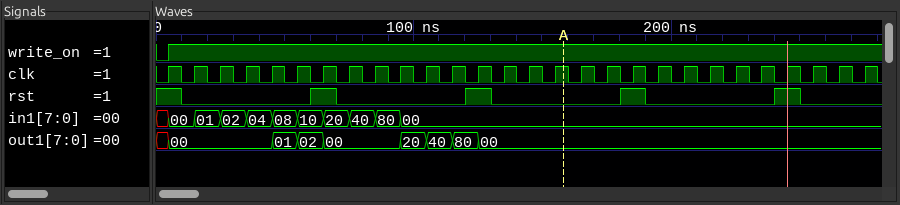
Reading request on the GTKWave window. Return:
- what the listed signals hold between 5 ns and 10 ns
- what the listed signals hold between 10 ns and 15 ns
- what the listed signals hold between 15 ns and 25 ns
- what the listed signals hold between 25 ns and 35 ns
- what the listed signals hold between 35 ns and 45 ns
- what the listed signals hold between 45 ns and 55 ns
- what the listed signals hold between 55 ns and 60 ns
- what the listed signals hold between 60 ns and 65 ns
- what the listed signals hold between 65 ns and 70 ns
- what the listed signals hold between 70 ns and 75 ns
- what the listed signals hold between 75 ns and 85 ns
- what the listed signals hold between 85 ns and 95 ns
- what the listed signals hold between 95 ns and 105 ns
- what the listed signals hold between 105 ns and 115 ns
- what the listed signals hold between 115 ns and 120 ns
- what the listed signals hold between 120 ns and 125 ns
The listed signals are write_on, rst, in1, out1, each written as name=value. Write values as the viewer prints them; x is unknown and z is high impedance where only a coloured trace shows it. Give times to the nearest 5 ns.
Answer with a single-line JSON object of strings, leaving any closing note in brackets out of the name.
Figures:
{"what the listed signals hold between 5 ns and 10 ns": "write_on=1, rst=1, in1=00, out1=00", "what the listed signals hold between 10 ns and 15 ns": "write_on=1, rst=0, in1=00, out1=00", "what the listed signals hold between 15 ns and 25 ns": "write_on=1, rst=0, in1=01, out1=00", "what the listed signals hold between 25 ns and 35 ns": "write_on=1, rst=0, in1=02, out1=00", "what the listed signals hold between 35 ns and 45 ns": "write_on=1, rst=0, in1=04, out1=00", "what the listed signals hold between 45 ns and 55 ns": "write_on=1, rst=0, in1=08, out1=01", "what the listed signals hold between 55 ns and 60 ns": "write_on=1, rst=0, in1=10, out1=02", "what the listed signals hold between 60 ns and 65 ns": "write_on=1, rst=1, in1=10, out1=02", "what the listed signals hold between 65 ns and 70 ns": "write_on=1, rst=1, in1=20, out1=00", "what the listed signals hold between 70 ns and 75 ns": "write_on=1, rst=0, in1=20, out1=00", "what the listed signals hold between 75 ns and 85 ns": "write_on=1, rst=0, in1=40, out1=00", "what the listed signals hold between 85 ns and 95 ns": "write_on=1, rst=0, in1=80, out1=00", "what the listed signals hold between 95 ns and 105 ns": "write_on=1, rst=0, in1=00, out1=20", "what the listed signals hold between 105 ns and 115 ns": "write_on=1, rst=0, in1=00, out1=40", "what the listed signals hold between 115 ns and 120 ns": "write_on=1, rst=0, in1=00, out1=80", "what the listed signals hold between 120 ns and 125 ns": "write_on=1, rst=1, in1=00, out1=80"}
